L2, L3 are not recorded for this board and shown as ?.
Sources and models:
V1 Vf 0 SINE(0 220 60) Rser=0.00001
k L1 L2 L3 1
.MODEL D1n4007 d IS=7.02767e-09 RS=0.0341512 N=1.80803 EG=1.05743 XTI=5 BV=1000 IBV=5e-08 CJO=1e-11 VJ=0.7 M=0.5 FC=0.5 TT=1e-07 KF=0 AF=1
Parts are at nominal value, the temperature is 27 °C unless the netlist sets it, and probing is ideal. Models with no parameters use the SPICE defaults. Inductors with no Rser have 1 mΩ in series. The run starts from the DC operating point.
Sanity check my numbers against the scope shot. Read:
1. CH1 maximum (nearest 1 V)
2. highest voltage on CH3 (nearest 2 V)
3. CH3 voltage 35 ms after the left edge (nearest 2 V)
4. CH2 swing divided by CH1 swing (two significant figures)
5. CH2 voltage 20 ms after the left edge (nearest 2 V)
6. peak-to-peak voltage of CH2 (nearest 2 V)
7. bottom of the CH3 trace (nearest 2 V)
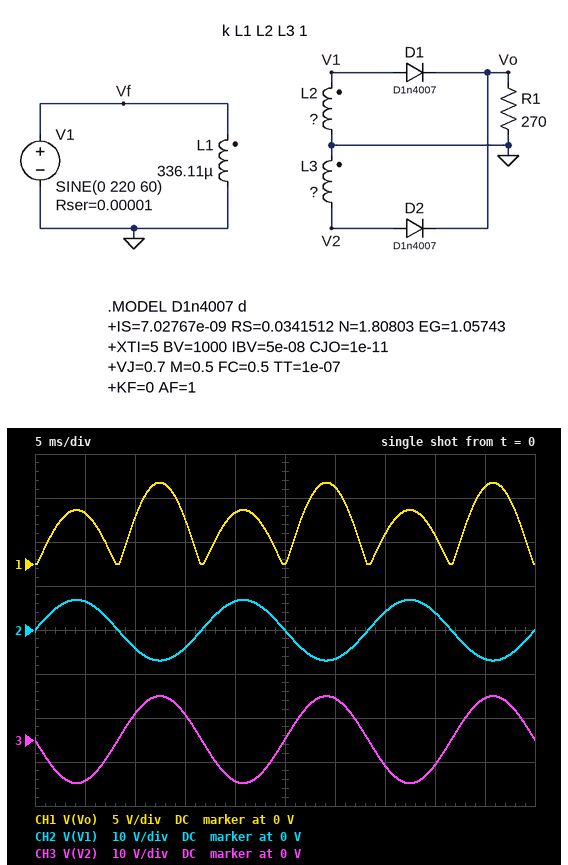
9 V
10 V
-6 V
1.5
6 V
14 V
-10 V
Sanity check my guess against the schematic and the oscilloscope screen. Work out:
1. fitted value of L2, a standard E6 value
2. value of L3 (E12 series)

330 nH
680 nH
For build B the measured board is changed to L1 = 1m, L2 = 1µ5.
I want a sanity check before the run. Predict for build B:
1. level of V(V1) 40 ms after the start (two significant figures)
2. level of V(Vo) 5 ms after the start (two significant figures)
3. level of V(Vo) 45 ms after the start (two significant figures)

5.0 V
7.4 V
4.8 V
